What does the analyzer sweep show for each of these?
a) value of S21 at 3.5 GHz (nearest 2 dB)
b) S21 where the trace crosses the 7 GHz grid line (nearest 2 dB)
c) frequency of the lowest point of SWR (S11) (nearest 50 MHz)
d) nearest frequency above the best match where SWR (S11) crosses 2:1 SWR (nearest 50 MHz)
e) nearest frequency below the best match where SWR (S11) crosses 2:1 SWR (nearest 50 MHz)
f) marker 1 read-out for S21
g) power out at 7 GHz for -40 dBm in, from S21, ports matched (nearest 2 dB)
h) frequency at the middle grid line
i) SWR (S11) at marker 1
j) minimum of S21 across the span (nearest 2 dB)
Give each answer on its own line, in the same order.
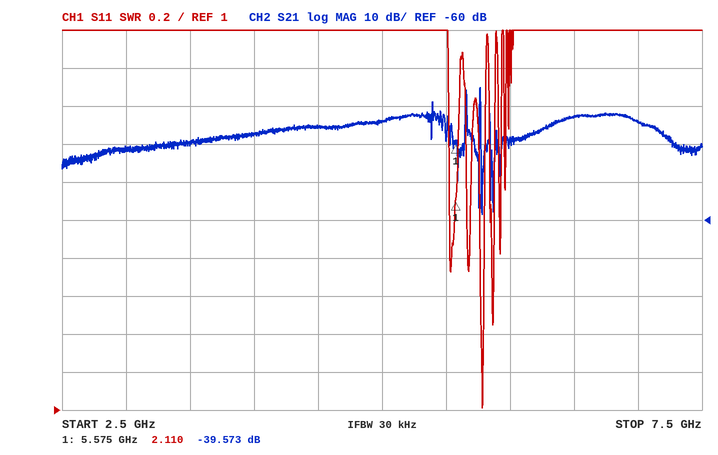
-40 dB
-34 dB
5.80 GHz
5.80 GHz
5.75 GHz
-39.573 dB
-74 dBm
5 GHz
2.110
-58 dB
